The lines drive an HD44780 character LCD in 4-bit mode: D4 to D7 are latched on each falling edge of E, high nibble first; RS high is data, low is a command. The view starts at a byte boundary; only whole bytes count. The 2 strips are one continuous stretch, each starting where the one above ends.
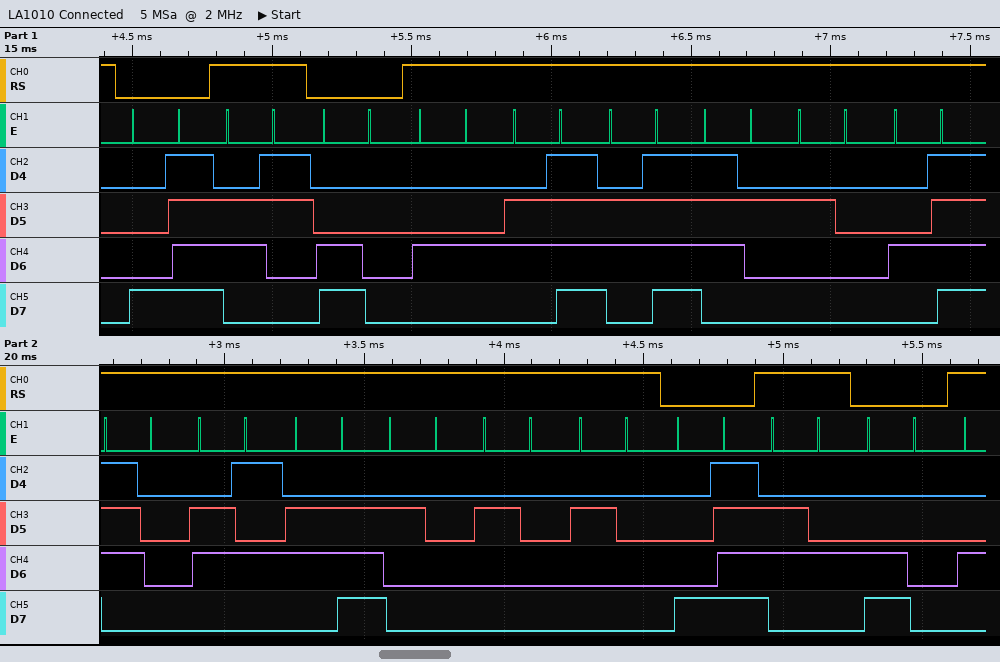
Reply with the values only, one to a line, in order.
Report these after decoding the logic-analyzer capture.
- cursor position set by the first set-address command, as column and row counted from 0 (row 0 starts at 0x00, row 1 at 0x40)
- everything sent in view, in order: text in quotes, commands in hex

column 15, row 0
0x8F "c" 0xC0 "Door Open   " 0x8F "d" 0xC0
